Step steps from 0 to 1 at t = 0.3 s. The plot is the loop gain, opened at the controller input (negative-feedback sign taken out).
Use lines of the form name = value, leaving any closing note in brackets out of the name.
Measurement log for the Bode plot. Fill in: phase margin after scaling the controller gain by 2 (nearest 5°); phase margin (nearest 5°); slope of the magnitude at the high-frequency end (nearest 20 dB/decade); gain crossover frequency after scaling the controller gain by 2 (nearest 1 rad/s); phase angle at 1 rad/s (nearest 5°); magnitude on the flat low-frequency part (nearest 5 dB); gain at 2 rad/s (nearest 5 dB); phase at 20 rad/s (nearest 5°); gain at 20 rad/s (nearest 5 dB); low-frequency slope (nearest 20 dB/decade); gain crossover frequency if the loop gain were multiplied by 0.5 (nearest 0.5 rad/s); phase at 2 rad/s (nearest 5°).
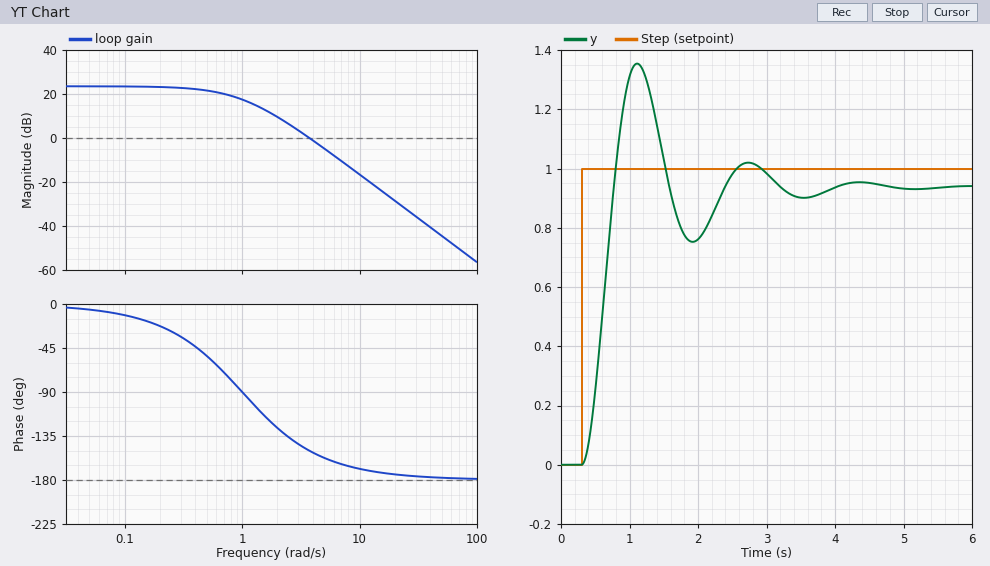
phase margin after scaling the controller gain by 2 = 20°
phase margin = 30°
slope of the magnitude at the high-frequency end = -40 dB/decade
gain crossover frequency after scaling the controller gain by 2 = 5 rad/s
phase angle at 1 rad/s = -90°
magnitude on the flat low-frequency part = 25 dB
gain at 2 rad/s = 10 dB
phase at 20 rad/s = -175°
gain at 20 rad/s = -30 dB
low-frequency slope = 0 dB/decade
gain crossover frequency if the loop gain were multiplied by 0.5 = 2.5 rad/s
phase at 2 rad/s = -125°
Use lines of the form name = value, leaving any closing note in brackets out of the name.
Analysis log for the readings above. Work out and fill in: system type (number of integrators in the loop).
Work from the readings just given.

system type = 0
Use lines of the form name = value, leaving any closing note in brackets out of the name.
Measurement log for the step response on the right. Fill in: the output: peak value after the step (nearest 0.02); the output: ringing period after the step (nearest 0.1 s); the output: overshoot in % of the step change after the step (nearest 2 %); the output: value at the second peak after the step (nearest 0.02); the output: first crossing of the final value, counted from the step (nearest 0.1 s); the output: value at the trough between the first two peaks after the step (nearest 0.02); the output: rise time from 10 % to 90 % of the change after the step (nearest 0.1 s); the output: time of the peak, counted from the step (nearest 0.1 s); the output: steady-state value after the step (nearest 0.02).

the output: peak value after the step = 1.36
the output: ringing period after the step = 1.6 s
the output: overshoot in % of the step change after the step = 44 %
the output: value at the second peak after the step = 1.02
the output: first crossing of the final value, counted from the step = 0.5 s
the output: value at the trough between the first two peaks after the step = 0.76
the output: rise time from 10 % to 90 % of the change after the step = 0.3 s
the output: time of the peak, counted from the step = 0.8 s
the output: steady-state value after the step = 0.94
